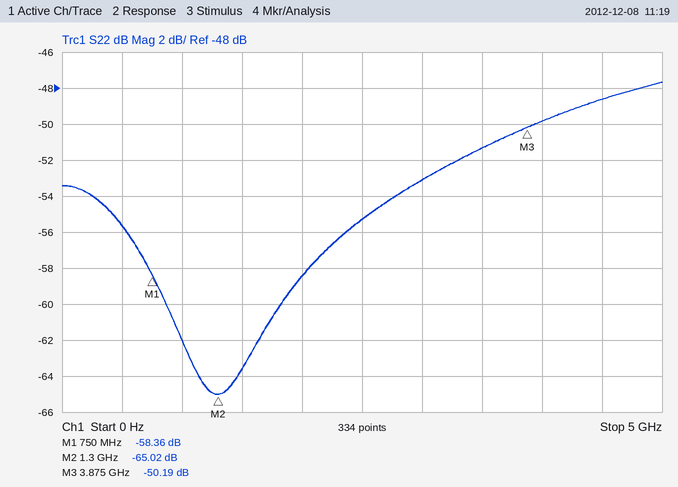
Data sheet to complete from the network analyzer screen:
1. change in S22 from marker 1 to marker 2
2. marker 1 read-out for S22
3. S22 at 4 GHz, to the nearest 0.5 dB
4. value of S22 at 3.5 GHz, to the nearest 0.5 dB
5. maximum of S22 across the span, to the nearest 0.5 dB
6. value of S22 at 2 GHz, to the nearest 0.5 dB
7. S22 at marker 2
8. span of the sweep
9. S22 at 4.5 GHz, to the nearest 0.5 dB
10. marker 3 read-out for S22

-6.66 dB
-58.36 dB
-50.0 dB
-51.5 dB
-47.5 dB
-58.5 dB
-65.02 dB
5 GHz
-48.5 dB
-50.19 dB
